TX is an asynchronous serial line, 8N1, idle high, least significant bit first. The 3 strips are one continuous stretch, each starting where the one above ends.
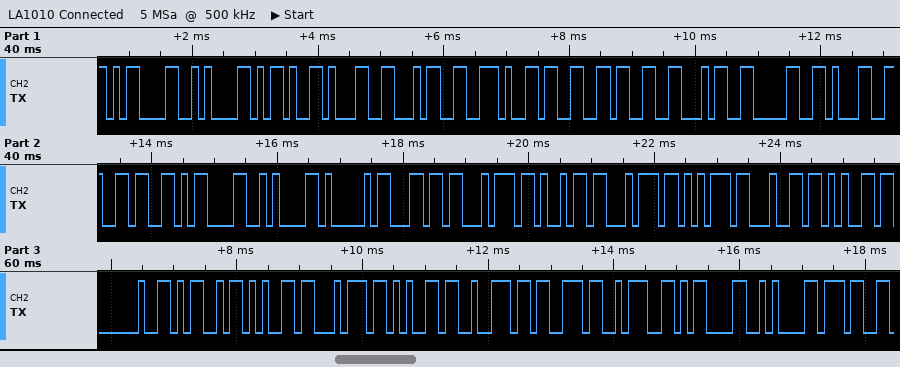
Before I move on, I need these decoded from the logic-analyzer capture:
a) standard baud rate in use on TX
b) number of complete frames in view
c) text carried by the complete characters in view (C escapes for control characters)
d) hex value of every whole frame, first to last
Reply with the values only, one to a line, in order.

9600 baud
33
"\r\n-14.334016\r\nAltitude Meters:\r\n7"
0D 0A 2D 31 34 2E 33 33 34 30 31 36 0D 0A 41 6C 74 69 74 75 64 65 20 4D 65 74 65 72 73 3A 0D 0A 37
